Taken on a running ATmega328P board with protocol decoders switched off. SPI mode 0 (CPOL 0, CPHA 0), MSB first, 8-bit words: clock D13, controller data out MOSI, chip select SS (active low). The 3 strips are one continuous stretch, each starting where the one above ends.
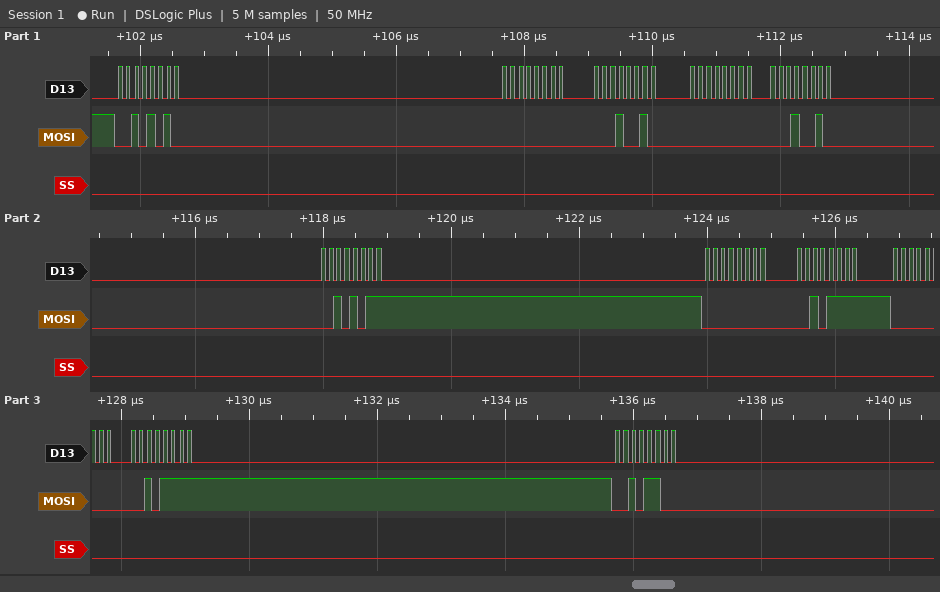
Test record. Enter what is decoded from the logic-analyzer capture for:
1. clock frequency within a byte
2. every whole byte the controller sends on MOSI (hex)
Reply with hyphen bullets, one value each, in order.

- 8 MHz
- 2A 00 12 00 12 2B 00 2F 00 2F 2C
